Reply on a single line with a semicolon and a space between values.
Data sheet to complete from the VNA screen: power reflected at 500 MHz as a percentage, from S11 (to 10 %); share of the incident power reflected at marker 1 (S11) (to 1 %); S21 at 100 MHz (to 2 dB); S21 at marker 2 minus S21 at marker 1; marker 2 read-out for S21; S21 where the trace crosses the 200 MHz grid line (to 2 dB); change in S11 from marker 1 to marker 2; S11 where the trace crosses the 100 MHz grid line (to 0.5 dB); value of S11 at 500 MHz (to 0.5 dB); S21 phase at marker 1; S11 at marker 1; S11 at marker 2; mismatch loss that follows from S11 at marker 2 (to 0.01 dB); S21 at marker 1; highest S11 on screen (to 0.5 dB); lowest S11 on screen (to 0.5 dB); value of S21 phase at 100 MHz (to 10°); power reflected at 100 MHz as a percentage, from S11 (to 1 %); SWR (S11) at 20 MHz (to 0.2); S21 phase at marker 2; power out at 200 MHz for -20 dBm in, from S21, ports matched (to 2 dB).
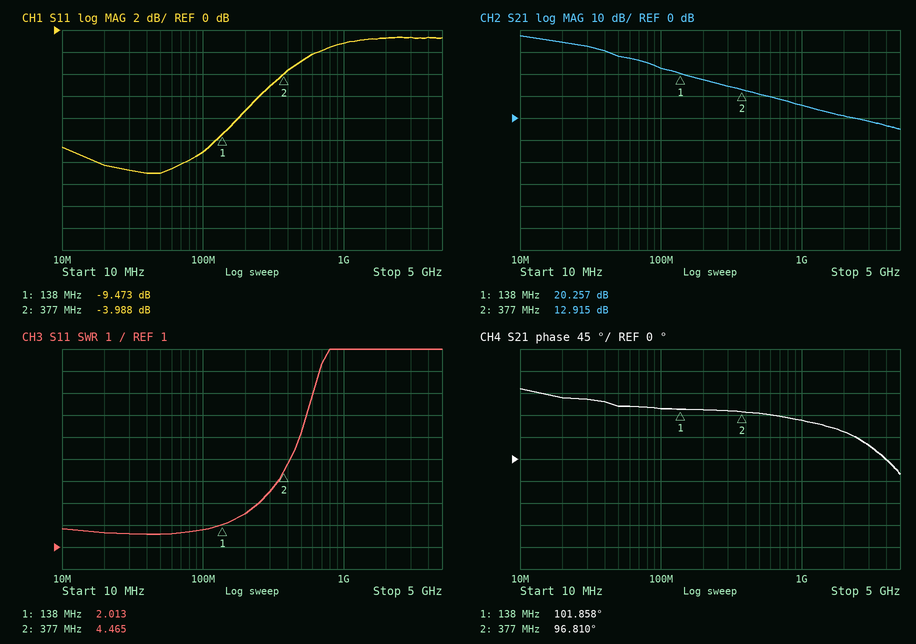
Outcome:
50 %; 11 %; 22 dB; -7.342 dB; 12.915 dB; 18 dB; 5.485 dB; -11.0 dB; -3.0 dB; 101.858°; -9.473 dB; -3.988 dB; 2.21 dB; 20.257 dB; -0.5 dB; -13.0 dB; 100°; 8 %; 1.6; 96.810°; -2 dBm
